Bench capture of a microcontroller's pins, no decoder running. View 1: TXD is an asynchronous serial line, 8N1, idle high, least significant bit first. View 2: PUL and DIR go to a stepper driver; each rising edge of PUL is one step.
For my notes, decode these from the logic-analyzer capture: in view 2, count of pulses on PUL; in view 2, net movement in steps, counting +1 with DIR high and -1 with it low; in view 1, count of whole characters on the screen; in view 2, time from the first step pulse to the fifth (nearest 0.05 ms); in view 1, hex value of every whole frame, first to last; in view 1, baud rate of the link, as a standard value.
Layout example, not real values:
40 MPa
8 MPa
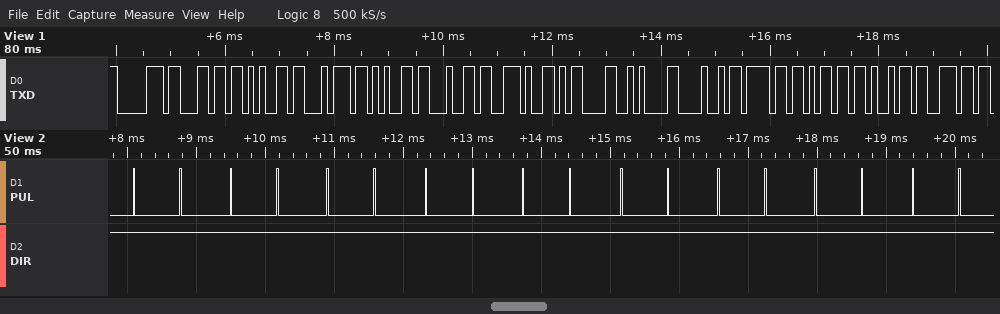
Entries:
18
+18
14
2.80 ms
0x70 0x6C 0x65 0x74 0x65 0x64 0x2E 0x0D 0x0A 0x48 0x6F 0x6D 0x69 0x6E
9600 baud
